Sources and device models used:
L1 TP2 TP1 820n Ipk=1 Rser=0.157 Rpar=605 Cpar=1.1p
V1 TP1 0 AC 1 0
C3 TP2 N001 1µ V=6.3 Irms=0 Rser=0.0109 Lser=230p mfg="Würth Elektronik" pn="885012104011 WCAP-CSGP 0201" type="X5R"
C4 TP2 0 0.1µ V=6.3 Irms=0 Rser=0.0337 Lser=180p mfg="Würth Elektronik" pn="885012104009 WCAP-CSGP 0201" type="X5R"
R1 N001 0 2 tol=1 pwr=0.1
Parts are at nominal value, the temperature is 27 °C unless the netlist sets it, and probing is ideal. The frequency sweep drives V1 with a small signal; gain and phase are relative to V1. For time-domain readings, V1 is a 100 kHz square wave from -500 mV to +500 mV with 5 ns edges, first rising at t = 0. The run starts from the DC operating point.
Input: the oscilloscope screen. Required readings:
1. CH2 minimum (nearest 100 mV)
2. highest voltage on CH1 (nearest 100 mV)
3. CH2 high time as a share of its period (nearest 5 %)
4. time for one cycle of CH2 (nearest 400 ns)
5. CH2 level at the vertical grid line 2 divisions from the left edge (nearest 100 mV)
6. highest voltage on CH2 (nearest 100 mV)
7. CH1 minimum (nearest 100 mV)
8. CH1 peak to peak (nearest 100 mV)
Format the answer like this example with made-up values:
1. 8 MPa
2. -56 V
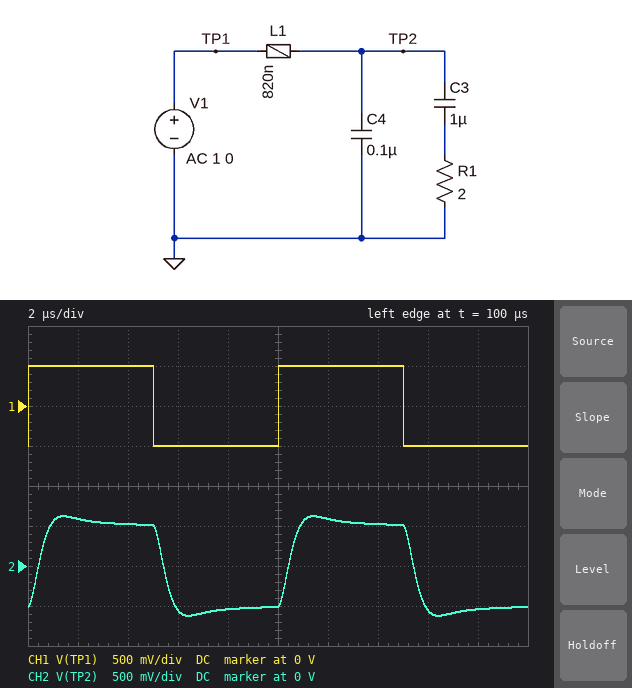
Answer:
1. -600 mV
2. 500 mV
3. 50 %
4. 10.0 µs
5. 500 mV
6. 600 mV
7. -500 mV
8. 1.0 V
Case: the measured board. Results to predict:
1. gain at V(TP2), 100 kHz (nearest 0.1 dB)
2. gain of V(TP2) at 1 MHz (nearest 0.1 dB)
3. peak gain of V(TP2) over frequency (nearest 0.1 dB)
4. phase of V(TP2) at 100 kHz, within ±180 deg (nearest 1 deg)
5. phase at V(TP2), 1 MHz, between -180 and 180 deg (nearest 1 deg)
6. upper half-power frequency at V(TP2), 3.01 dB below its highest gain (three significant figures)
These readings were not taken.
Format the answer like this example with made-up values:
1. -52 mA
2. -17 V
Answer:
1. 0.8 dB
2. -11.1 dB
3. 0.9 dB
4. -13 deg
5. -130 deg
6. 479 kHz
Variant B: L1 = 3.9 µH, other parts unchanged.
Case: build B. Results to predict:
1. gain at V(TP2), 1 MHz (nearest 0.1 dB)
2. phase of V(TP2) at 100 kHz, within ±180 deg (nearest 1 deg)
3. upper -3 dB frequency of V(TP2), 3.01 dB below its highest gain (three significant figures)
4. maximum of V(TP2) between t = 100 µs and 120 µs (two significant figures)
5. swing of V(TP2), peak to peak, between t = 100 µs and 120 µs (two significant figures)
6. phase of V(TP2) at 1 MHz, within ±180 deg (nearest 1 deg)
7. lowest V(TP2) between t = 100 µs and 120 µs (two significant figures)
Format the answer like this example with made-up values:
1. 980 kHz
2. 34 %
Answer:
1. -25.9 dB
2. -69 deg
3. 110 kHz
4. 780 mV
5. 1.6 V
6. -138 deg
7. -780 mV
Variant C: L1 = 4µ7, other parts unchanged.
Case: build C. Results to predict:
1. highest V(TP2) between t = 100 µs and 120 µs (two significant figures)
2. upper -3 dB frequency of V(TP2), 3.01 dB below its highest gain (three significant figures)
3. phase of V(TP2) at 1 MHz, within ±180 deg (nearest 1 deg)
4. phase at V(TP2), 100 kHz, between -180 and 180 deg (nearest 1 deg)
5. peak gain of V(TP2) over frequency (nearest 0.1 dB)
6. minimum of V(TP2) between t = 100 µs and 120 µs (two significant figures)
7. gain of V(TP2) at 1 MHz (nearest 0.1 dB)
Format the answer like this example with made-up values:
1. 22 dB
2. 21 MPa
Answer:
1. 720 mV
2. 96.5 kHz
3. -138 deg
4. -81 deg
5. 3.8 dB
6. -720 mV
7. -27.6 dB
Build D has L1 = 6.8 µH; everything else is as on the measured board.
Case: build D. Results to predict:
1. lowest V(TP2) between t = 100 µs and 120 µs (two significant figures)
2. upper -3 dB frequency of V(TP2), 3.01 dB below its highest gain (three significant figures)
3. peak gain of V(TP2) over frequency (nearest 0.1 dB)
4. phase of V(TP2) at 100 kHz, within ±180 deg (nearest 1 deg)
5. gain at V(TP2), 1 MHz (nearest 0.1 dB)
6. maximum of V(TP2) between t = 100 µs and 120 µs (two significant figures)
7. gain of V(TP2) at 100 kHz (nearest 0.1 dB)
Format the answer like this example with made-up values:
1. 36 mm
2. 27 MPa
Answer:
1. -510 mV
2. 75.6 kHz
3. 4.7 dB
4. -100 deg
5. -30.9 dB
6. 510 mV
7. -2.8 dB
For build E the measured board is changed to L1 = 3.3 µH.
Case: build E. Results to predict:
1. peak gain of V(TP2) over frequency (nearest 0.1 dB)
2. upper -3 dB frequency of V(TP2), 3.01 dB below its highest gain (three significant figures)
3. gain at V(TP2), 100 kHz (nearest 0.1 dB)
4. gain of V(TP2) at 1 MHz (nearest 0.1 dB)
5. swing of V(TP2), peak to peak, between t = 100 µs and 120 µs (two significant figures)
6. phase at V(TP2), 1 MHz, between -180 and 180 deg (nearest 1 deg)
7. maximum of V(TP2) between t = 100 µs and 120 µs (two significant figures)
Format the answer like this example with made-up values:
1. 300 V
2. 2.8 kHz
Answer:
1. 3.0 dB
2. 125 kHz
3. 1.9 dB
4. -24.4 dB
5. 1.6 V
6. -138 deg
7. 780 mV
